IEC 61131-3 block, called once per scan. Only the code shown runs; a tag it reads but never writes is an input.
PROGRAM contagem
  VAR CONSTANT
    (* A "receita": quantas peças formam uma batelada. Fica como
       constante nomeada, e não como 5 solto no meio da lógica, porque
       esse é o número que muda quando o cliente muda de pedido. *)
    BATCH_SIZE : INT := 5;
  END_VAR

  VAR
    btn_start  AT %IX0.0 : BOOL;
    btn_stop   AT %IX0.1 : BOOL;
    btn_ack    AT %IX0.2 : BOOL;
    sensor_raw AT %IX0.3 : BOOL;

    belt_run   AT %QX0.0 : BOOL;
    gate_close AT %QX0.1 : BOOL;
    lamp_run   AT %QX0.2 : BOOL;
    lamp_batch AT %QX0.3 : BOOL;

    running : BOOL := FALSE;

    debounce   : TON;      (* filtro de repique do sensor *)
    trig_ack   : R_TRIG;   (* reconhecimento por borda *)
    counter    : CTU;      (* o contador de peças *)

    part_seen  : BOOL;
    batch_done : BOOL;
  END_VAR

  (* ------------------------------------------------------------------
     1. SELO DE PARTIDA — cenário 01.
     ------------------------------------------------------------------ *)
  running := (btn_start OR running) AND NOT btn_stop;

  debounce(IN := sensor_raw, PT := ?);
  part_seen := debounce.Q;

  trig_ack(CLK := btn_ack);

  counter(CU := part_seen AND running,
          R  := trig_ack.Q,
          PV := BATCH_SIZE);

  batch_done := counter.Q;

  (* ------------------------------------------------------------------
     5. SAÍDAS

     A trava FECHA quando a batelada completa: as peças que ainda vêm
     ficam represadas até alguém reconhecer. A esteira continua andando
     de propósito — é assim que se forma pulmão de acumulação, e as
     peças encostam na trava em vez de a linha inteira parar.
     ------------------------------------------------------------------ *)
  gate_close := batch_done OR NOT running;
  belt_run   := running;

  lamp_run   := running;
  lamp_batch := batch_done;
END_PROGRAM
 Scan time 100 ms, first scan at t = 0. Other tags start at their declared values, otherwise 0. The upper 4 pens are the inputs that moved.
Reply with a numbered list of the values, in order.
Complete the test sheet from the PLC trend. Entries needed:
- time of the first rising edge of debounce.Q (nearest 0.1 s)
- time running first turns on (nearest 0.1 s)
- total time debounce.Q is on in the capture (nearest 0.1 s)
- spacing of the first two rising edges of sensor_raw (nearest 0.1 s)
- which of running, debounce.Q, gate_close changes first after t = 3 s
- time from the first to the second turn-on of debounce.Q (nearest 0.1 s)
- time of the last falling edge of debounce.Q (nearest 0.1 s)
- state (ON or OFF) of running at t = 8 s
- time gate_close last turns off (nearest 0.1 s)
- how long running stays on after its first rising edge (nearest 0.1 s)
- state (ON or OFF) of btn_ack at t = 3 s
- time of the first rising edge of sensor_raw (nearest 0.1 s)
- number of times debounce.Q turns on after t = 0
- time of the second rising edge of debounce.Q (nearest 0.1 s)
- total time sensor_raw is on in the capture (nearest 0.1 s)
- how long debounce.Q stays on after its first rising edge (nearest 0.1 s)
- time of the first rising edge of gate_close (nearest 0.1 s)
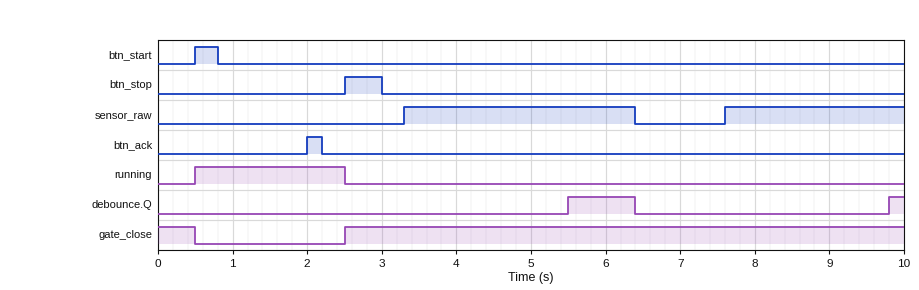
1. 5.5 s
2. 0.5 s
3. 1.1 s
4. 4.3 s
5. debounce.Q
6. 4.3 s
7. 6.4 s
8. OFF
9. 0.5 s
10. 2.0 s
11. OFF
12. 3.3 s
13. 2
14. 9.8 s
15. 5.5 s
16. 0.9 s
17. 2.5 s
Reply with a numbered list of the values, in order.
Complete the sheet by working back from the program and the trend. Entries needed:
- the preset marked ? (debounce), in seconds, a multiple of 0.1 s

1. 2.2 s
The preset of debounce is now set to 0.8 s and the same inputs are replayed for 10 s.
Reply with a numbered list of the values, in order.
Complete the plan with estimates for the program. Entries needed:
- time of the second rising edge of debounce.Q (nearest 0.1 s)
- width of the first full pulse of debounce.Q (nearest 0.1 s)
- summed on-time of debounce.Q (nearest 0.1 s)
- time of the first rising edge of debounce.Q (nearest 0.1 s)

1. 8.4 s
2. 2.3 s
3. 3.9 s
4. 4.1 s
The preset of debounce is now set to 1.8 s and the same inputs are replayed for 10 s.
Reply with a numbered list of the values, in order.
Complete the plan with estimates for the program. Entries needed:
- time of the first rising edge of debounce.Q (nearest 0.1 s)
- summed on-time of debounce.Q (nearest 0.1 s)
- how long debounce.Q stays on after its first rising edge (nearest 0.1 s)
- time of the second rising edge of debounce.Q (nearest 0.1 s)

1. 5.1 s
2. 1.9 s
3. 1.3 s
4. 9.4 s
